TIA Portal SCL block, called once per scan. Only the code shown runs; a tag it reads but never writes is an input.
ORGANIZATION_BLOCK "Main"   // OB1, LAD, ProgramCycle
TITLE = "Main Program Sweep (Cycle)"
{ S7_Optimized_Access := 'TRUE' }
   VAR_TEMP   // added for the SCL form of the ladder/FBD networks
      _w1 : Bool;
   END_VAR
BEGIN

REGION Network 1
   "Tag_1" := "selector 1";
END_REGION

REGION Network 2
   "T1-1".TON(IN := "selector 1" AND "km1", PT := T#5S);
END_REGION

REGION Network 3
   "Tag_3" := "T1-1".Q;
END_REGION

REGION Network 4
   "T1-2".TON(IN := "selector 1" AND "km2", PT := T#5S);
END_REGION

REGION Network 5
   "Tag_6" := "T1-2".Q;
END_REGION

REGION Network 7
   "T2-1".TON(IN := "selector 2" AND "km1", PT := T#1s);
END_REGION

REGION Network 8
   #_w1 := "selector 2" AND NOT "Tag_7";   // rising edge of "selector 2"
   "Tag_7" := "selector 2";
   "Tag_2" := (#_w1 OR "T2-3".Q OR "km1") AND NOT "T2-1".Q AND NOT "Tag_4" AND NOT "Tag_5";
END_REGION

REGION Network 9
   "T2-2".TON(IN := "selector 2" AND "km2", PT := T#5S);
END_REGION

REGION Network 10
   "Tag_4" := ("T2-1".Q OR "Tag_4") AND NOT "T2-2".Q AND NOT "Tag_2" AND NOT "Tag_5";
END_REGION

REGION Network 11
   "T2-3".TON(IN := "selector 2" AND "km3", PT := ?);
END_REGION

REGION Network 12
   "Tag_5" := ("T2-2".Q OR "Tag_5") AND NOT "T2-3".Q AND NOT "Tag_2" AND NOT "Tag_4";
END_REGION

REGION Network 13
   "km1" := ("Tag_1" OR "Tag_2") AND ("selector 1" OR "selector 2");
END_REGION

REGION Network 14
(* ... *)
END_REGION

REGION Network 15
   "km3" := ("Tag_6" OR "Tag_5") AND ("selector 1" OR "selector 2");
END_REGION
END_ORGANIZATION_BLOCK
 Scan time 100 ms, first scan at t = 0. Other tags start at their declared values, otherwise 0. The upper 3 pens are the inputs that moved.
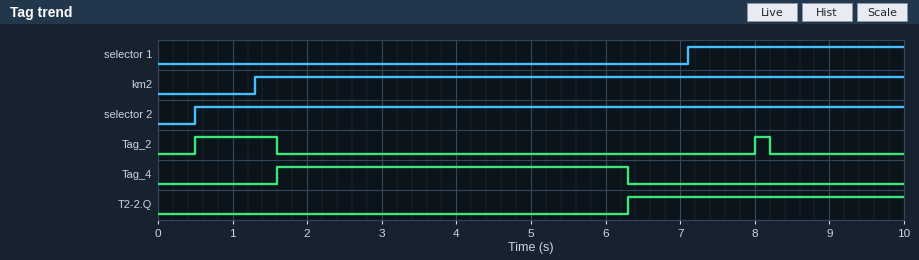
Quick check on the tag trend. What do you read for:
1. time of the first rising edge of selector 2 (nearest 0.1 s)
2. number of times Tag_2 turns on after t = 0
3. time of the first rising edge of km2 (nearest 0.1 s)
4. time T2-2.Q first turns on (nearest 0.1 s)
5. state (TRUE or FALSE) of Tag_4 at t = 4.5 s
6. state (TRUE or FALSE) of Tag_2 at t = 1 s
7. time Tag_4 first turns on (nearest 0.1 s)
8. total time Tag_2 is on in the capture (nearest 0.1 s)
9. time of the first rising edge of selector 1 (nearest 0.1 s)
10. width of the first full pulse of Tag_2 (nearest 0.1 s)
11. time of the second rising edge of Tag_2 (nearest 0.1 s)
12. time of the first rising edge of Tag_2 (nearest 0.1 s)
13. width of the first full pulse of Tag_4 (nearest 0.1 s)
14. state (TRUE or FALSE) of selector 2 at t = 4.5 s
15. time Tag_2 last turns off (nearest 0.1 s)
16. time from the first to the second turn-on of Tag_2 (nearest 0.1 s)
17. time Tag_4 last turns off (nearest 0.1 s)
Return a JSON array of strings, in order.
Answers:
["0.5 s", "2", "1.3 s", "6.3 s", "TRUE", "TRUE", "1.6 s", "1.3 s", "7.1 s", "1.1 s", "8.0 s", "0.5 s", "4.7 s", "TRUE", "8.2 s", "7.5 s", "6.3 s"]
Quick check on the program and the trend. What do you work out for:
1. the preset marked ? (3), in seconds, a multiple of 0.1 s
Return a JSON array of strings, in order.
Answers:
["1.5 s"]
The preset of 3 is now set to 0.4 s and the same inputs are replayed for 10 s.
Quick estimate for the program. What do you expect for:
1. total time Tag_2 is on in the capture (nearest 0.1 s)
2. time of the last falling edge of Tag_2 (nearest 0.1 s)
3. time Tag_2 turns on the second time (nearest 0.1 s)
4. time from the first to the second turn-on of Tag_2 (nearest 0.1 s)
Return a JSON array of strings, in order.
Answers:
["2.2 s", "8.0 s", "6.9 s", "6.4 s"]
